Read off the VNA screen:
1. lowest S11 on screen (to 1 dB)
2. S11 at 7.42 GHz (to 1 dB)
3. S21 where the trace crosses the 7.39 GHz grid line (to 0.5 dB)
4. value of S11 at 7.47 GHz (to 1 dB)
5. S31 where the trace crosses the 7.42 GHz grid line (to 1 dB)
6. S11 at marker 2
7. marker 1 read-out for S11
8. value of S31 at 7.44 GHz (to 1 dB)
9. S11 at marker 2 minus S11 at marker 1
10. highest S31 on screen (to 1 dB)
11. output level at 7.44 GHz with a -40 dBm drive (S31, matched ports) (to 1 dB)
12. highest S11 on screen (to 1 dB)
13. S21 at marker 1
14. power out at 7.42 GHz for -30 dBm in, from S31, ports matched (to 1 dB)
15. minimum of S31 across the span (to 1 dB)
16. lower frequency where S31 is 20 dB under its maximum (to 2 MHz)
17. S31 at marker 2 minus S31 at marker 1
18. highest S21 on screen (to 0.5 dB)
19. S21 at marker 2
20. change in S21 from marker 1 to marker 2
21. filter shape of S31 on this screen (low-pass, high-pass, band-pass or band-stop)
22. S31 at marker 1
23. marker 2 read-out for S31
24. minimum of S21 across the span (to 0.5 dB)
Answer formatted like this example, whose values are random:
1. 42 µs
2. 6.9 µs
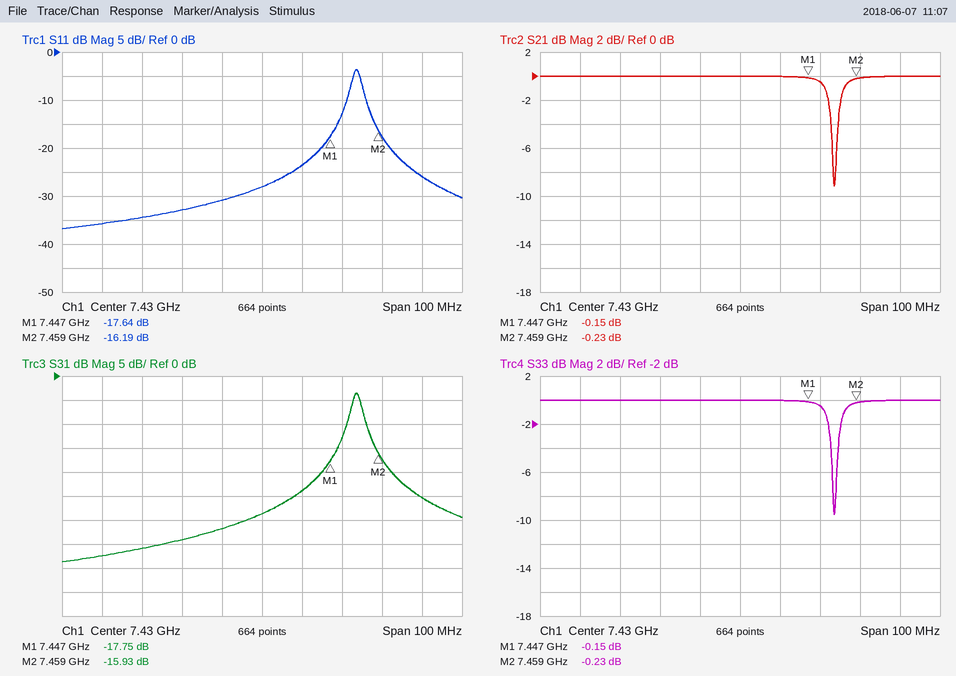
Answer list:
1. -37 dB
2. -31 dB
3. 0.0 dB
4. -26 dB
5. -32 dB
6. -16.19 dB
7. -17.64 dB
8. -24 dB
9. 1.45 dB
10. -4 dB
11. -64 dBm
12. -4 dB
13. -0.15 dB
14. -62 dBm
15. -39 dB
16. 7.440 GHz
17. 1.82 dB
18. 0.0 dB
19. -0.23 dB
20. -0.08 dB
21. band-pass
22. -17.75 dB
23. -15.93 dB
24. -9.0 dB
